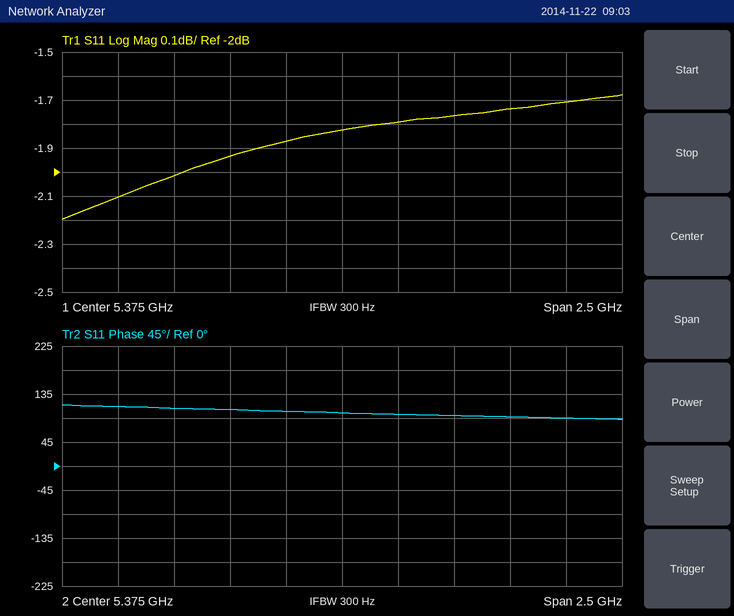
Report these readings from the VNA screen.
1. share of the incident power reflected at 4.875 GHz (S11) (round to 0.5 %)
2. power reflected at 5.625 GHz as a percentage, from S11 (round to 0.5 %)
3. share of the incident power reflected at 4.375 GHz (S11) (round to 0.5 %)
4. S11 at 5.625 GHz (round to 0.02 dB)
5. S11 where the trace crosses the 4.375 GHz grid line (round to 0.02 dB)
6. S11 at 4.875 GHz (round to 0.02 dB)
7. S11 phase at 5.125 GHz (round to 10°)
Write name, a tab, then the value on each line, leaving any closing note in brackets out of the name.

share of the incident power reflected at 4.875 GHz (S11)	64.0 %
power reflected at 5.625 GHz as a percentage, from S11	66.0 %
share of the incident power reflected at 4.375 GHz (S11)	61.5 %
S11 at 5.625 GHz	-1.80 dB
S11 where the trace crosses the 4.375 GHz grid line	-2.10 dB
S11 at 4.875 GHz	-1.94 dB
S11 phase at 5.125 GHz	100°
